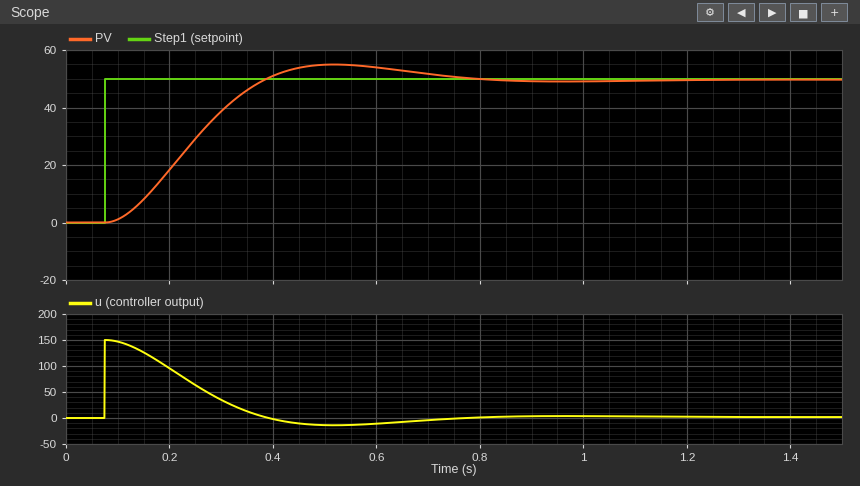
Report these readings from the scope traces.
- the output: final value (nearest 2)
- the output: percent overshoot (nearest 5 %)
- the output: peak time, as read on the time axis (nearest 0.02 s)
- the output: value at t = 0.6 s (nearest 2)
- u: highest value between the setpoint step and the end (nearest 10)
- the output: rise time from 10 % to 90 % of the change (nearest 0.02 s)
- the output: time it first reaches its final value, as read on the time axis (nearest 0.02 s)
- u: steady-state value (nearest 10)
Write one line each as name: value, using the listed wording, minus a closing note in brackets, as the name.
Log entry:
the output: final value: 50
the output: percent overshoot: 10 %
the output: peak time, as read on the time axis: 0.52 s
the output: value at t = 0.6 s: 54
u: highest value between the setpoint step and the end: 150
the output: rise time from 10 % to 90 % of the change: 0.20 s
the output: time it first reaches its final value, as read on the time axis: 0.38 s
u: steady-state value: 0
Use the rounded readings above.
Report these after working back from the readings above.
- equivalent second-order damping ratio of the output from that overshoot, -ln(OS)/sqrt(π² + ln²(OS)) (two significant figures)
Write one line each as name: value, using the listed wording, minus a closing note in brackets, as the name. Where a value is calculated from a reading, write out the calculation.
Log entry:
equivalent second-order damping ratio of the output from that overshoot, -ln(OS)/sqrt(π² + ln²(OS)): ln(0.1) = -2.303; 2.303 / sqrt(9.870 + 5.302) = 0.59
